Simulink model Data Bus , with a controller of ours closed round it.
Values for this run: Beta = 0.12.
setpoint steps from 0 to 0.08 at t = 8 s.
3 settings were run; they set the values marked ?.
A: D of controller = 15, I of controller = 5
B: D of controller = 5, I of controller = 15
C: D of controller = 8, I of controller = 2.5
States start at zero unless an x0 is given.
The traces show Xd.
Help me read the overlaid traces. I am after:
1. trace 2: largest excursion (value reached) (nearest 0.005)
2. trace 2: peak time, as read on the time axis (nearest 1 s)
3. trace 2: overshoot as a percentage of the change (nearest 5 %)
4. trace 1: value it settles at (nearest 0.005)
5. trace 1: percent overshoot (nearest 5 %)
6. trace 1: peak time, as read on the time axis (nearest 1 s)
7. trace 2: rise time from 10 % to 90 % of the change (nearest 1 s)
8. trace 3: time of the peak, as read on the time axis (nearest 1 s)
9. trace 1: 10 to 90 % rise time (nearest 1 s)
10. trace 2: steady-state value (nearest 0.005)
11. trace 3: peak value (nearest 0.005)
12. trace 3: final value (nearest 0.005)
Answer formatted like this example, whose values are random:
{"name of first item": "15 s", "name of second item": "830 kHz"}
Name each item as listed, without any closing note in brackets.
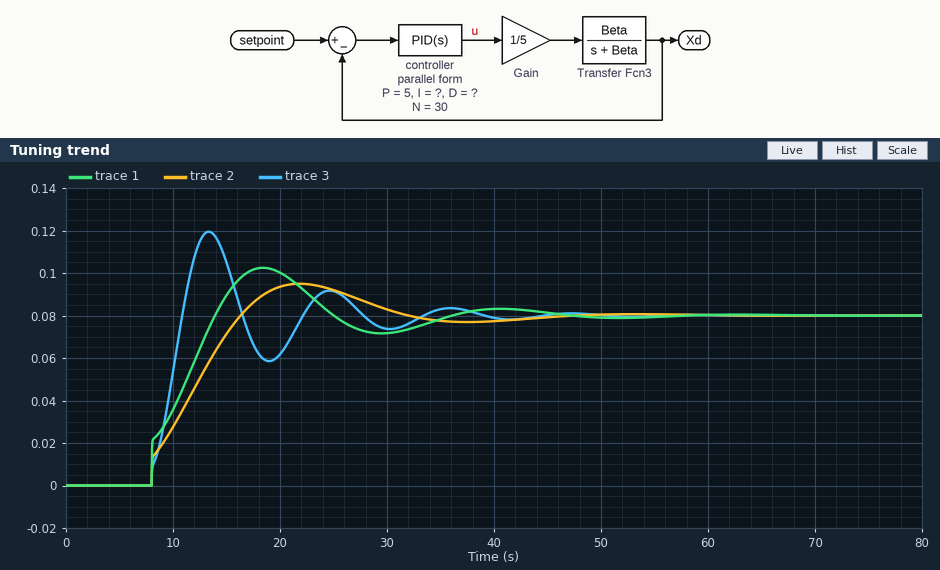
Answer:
{"trace 2: largest excursion (value reached)": "0.095", "trace 2: peak time, as read on the time axis": "22 s", "trace 2: overshoot as a percentage of the change": "20 %", "trace 1: value it settles at": "0.080", "trace 1: percent overshoot": "30 %", "trace 1: peak time, as read on the time axis": "18 s", "trace 2: rise time from 10 % to 90 % of the change": "7 s", "trace 3: time of the peak, as read on the time axis": "13 s", "trace 1: 10 to 90 % rise time": "5 s", "trace 2: steady-state value": "0.080", "trace 3: peak value": "0.120", "trace 3: final value": "0.080"}
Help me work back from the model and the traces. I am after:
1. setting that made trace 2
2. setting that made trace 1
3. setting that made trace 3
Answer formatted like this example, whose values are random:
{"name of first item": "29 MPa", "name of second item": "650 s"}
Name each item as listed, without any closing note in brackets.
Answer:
{"setting that made trace 2": "C", "setting that made trace 1": "A", "setting that made trace 3": "B"}
